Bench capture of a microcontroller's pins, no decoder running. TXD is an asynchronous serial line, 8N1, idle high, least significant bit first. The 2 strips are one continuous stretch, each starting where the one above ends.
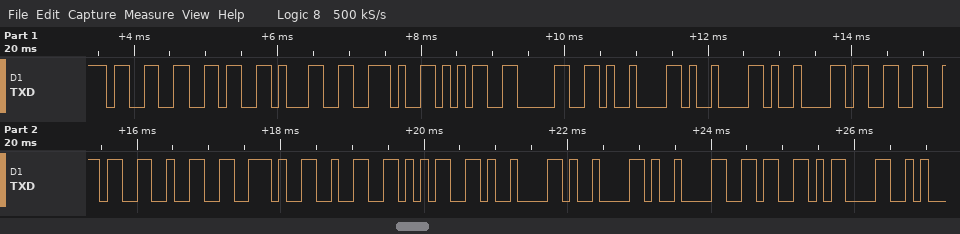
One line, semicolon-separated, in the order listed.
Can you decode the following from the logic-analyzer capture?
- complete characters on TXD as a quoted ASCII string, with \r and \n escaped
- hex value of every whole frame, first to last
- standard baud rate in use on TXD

"361.50\t\t\t362.25\t\t\t6\r"; 0x33 0x36 0x31 0x2E 0x35 0x30 0x09 0x09 0x09 0x33 0x36 0x32 0x2E 0x32 0x35 0x09 0x09 0x09 0x36 0x0D; 9600 baud
